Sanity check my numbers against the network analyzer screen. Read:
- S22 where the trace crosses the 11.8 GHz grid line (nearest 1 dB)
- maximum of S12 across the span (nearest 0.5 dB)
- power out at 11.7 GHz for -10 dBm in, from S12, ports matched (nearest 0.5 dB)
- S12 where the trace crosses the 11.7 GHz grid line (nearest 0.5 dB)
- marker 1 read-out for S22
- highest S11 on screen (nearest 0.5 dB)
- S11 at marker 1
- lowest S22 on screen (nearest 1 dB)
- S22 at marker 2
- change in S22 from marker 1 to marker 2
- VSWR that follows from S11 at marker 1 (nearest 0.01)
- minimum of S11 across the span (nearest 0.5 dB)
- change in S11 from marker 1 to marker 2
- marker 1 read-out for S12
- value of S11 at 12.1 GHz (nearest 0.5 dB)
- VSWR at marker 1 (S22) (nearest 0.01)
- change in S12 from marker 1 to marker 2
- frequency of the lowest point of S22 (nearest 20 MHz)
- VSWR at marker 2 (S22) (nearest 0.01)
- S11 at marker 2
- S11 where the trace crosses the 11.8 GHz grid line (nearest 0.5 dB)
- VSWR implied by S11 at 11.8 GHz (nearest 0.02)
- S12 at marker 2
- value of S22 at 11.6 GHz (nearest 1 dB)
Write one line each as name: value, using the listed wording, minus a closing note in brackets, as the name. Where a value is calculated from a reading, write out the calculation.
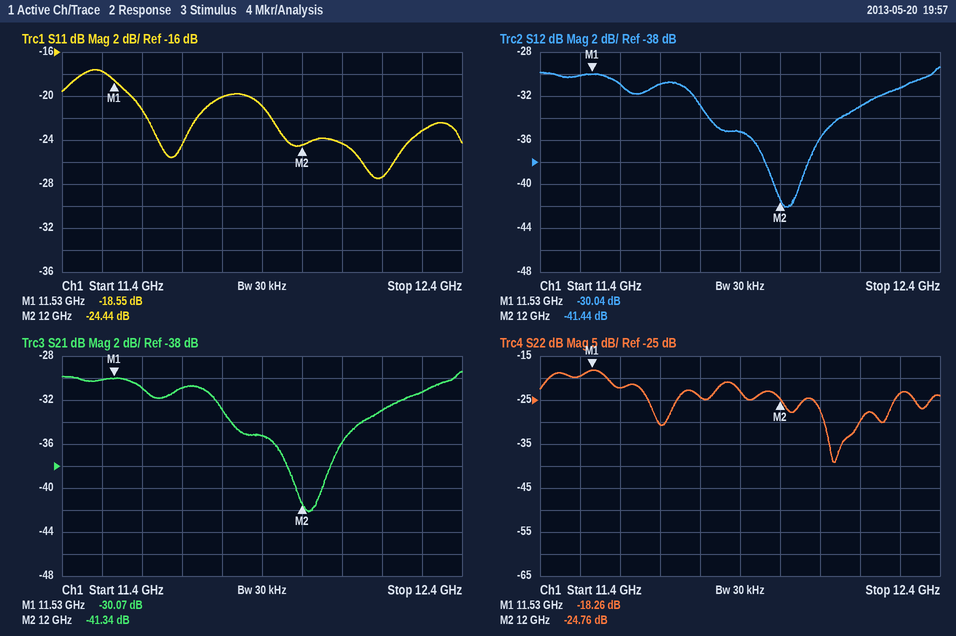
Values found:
S22 where the trace crosses the 11.8 GHz grid line: -24 dB
maximum of S12 across the span: -29.5 dB
power out at 11.7 GHz for -10 dBm in, from S12, ports matched: -10 dBm + (-31.0 dB) = -41.0 dBm
S12 where the trace crosses the 11.7 GHz grid line: -31.0 dB
marker 1 read-out for S22: -18.26 dB
highest S11 on screen: -17.5 dB
S11 at marker 1: -18.55 dB
lowest S22 on screen: -39 dB
S22 at marker 2: -24.76 dB
change in S22 from marker 1 to marker 2: -24.76 − (-18.26) = -6.50 dB
VSWR that follows from S11 at marker 1: (1 + 0.1182)/(1 − 0.1182) ≈ 1.27
minimum of S11 across the span: -27.5 dB
change in S11 from marker 1 to marker 2: -24.44 − (-18.55) = -5.89 dB
marker 1 read-out for S12: -30.04 dB
value of S11 at 12.1 GHz: -24.5 dB
VSWR at marker 1 (S22): (1 + 0.1222)/(1 − 0.1222) ≈ 1.28
change in S12 from marker 1 to marker 2: -41.44 − (-30.04) = -11.40 dB
frequency of the lowest point of S22: 12.14 GHz
VSWR at marker 2 (S22): (1 + 0.0578)/(1 − 0.0578) ≈ 1.12
S11 at marker 2: -24.44 dB
S11 where the trace crosses the 11.8 GHz grid line: -20.0 dB
VSWR implied by S11 at 11.8 GHz: |Γ| = 10^(-20/20) = 0.1000; VSWR = (1 + 0.1000)/(1 − 0.1000) ≈ 1.22
S12 at marker 2: -41.44 dB
value of S22 at 11.6 GHz: -22 dB
